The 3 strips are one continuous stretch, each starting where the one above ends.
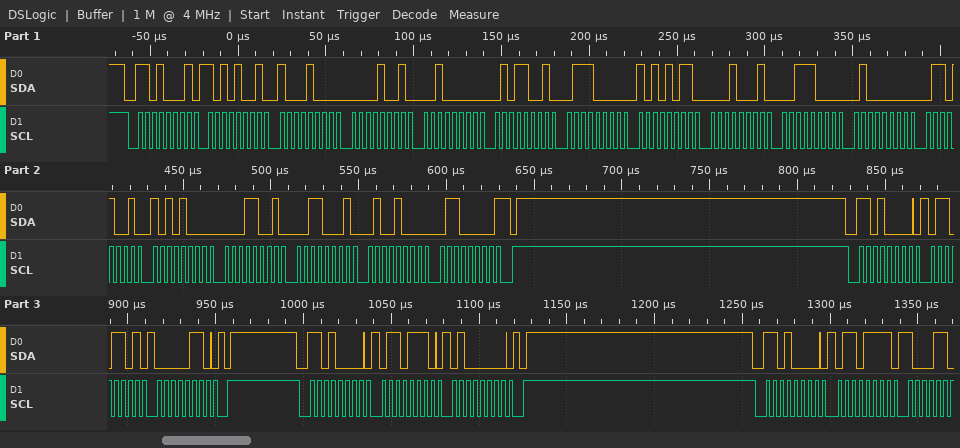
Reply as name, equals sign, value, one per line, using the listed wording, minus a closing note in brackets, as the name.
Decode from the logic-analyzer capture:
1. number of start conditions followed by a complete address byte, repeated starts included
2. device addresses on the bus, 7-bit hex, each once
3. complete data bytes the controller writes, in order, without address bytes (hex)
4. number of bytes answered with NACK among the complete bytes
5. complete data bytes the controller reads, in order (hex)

number of start conditions followed by a complete address byte, repeated starts included = 4
device addresses on the bus, 7-bit hex, each once = 0x68
complete data bytes the controller writes, in order, without address bytes = 6D 06 6E 40 6F
number of bytes answered with NACK among the complete bytes = 1
complete data bytes the controller reads, in order = A9 88 09 20 59 70 AB 11 38 40 69 A8 19 31 48 60
